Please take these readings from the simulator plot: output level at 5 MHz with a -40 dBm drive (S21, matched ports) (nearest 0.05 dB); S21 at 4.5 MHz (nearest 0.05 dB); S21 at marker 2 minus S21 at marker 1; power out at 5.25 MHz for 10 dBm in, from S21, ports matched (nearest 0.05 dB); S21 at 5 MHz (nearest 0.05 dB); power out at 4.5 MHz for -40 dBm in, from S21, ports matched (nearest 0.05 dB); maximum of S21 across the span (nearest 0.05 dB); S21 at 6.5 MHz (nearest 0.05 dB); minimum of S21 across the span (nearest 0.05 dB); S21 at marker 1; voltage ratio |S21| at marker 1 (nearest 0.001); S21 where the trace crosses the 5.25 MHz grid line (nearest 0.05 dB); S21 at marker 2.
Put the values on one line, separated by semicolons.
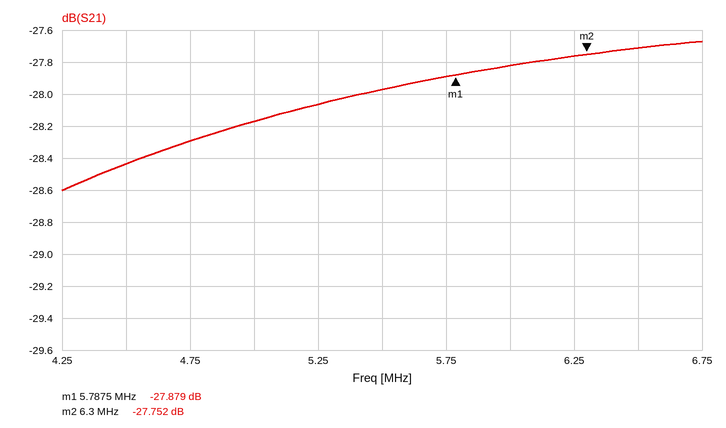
-68.15 dBm; -28.45 dB; 0.127 dB; -18.05 dBm; -28.15 dB; -68.45 dBm; -27.65 dB; -27.70 dB; -28.60 dB; -27.879 dB; 0.040; -28.05 dB; -27.752 dB
